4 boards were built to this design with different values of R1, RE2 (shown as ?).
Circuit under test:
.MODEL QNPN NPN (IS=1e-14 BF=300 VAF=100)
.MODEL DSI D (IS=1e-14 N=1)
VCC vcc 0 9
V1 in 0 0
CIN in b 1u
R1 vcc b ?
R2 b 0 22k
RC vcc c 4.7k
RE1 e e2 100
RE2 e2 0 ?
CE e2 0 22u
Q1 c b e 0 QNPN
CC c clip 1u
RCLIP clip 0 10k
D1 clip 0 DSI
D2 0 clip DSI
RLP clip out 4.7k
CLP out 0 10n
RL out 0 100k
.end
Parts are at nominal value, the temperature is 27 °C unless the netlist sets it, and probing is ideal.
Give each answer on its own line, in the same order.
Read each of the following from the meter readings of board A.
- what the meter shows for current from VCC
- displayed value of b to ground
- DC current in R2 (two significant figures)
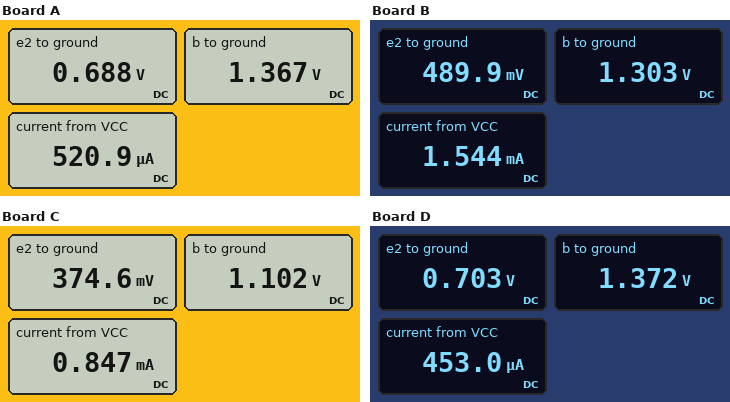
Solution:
520.9 µA
1.367 V
62 µA
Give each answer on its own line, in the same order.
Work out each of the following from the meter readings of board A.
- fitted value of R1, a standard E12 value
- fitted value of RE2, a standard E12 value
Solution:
120 kΩ
1.5 kΩ
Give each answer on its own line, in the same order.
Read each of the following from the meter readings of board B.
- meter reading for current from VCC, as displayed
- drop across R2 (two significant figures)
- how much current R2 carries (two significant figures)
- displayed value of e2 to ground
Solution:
1.544 mA
1.3 V
59 µA
489.9 mV
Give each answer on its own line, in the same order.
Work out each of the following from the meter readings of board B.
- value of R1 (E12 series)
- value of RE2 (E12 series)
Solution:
120 kΩ
330 Ω
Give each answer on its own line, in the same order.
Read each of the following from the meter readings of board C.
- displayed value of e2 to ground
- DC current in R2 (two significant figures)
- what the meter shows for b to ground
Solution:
374.6 mV
50 µA
1.102 V
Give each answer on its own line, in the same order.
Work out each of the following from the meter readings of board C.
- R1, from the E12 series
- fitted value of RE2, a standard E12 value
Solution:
150 kΩ
470 Ω
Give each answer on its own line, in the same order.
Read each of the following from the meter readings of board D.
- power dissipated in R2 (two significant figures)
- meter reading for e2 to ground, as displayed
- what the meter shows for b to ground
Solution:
86 µW
0.703 V
1.372 V
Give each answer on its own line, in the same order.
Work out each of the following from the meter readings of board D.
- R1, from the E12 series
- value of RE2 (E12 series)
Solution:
120 kΩ
1.8 kΩ
